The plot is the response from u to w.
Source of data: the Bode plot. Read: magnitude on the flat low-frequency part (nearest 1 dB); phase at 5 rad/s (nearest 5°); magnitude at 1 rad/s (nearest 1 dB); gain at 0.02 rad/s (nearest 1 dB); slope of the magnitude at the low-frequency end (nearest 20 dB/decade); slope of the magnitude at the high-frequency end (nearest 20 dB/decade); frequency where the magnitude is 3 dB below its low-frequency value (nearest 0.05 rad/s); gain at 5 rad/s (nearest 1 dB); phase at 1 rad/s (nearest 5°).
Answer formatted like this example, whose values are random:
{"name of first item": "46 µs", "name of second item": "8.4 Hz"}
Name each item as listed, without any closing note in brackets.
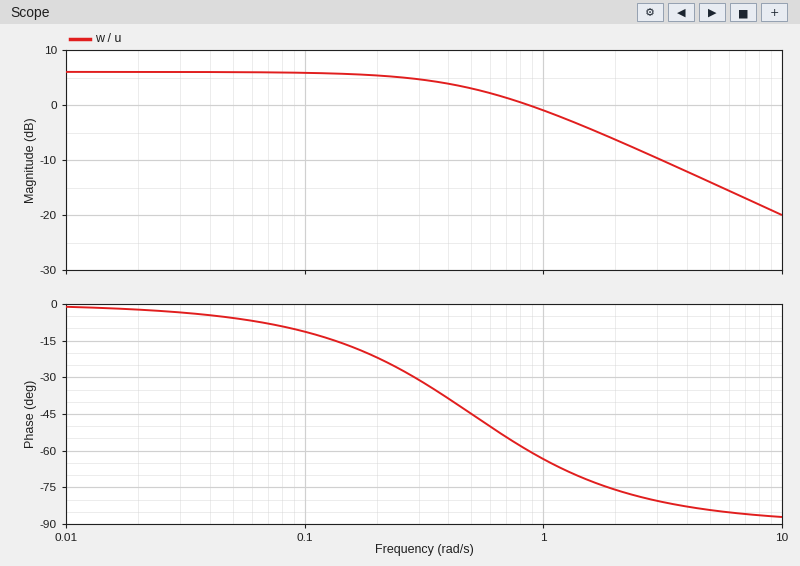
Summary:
{"magnitude on the flat low-frequency part": "6 dB", "phase at 5 rad/s": "-85°", "magnitude at 1 rad/s": "-1 dB", "gain at 0.02 rad/s": "6 dB", "slope of the magnitude at the low-frequency end": "0 dB/decade", "slope of the magnitude at the high-frequency end": "-20 dB/decade", "frequency where the magnitude is 3 dB below its low-frequency value": "0.50 rad/s", "gain at 5 rad/s": "-14 dB", "phase at 1 rad/s": "-65°"}
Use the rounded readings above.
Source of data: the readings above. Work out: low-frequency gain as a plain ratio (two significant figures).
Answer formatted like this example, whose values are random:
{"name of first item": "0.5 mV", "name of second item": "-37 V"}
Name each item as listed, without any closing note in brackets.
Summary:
{"low-frequency gain as a plain ratio": "2.0"}
